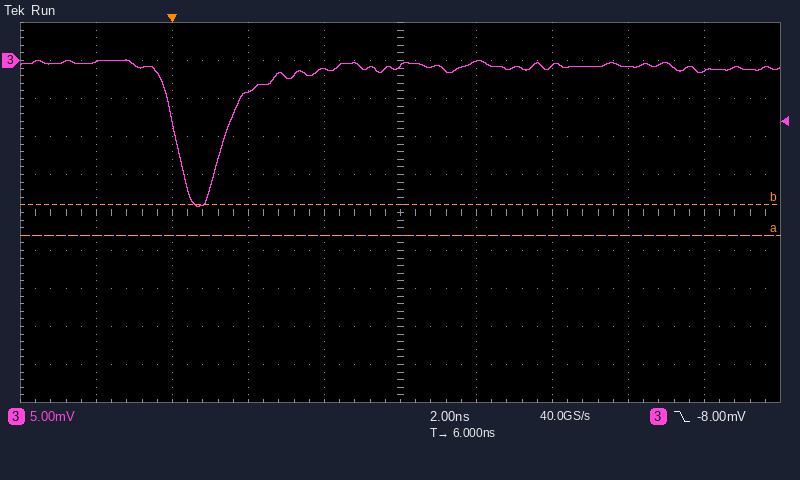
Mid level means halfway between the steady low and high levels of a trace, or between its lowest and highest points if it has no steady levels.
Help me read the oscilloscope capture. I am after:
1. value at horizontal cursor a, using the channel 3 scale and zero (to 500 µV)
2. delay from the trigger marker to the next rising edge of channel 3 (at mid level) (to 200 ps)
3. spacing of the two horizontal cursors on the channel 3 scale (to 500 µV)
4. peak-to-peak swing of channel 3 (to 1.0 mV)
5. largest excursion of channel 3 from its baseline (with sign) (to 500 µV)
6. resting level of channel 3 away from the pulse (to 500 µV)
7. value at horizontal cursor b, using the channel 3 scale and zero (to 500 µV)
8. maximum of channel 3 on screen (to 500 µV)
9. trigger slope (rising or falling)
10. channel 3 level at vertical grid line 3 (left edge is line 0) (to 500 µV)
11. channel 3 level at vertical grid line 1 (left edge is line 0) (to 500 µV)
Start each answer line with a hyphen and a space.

- -23.0 mV
- 1.4 ns
- 4.0 mV
- 19.0 mV
- -18.5 mV
- -1.0 mV
- -19.0 mV
- 0.0 mV
- falling
- -4.0 mV
- 0.0 mV
